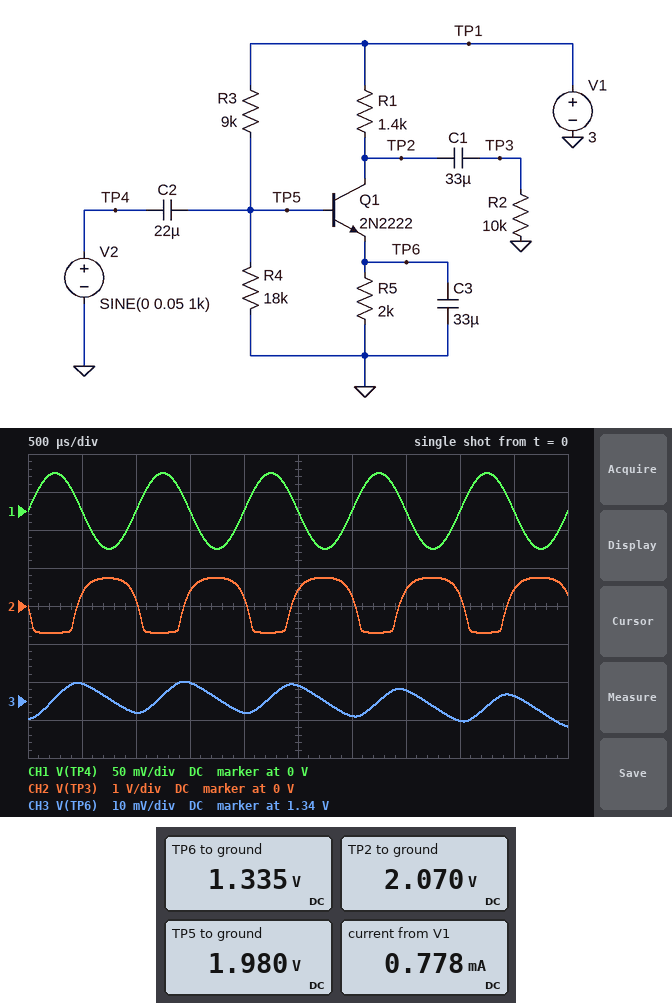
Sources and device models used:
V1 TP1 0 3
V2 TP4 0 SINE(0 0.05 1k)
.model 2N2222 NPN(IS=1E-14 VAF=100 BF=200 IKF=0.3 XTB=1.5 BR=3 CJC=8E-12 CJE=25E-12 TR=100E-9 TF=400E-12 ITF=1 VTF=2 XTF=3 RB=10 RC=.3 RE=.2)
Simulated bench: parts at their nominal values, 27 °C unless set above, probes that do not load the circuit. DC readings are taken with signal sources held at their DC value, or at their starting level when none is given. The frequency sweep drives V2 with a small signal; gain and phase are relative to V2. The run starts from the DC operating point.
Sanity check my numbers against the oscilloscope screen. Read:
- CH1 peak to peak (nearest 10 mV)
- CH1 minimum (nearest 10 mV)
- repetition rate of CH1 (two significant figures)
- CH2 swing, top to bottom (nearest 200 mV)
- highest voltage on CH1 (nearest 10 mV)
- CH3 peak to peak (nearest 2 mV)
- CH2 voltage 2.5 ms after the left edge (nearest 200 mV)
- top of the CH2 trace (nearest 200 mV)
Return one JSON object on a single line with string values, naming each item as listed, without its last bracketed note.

{"CH1 peak to peak": "100 mV", "CH1 minimum": "-50 mV", "repetition rate of CH1": "1.0 kHz", "CH2 swing, top to bottom": "1.4 V", "highest voltage on CH1": "50 mV", "CH3 peak to peak": "12 mV", "CH2 voltage 2.5 ms after the left edge": "400 mV", "top of the CH2 trace": "800 mV"}
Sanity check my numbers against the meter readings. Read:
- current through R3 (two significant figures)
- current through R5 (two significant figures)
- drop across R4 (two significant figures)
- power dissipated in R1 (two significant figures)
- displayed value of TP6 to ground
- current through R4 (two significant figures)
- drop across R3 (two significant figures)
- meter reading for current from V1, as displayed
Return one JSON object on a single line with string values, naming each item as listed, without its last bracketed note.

{"current through R3": "110 µA", "current through R5": "670 µA", "drop across R4": "2.0 V", "power dissipated in R1": "620 µW", "displayed value of TP6 to ground": "1.335 V", "current through R4": "110 µA", "drop across R3": "1.0 V", "meter reading for current from V1, as displayed": "0.778 mA"}
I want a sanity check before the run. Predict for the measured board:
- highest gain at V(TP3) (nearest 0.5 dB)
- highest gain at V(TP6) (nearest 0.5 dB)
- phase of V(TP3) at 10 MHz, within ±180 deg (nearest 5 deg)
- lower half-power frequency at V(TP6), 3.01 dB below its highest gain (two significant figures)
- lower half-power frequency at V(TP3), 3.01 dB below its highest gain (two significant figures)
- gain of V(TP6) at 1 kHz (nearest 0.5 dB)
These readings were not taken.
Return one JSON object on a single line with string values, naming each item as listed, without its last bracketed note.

{"highest gain at V(TP3)": "30.0 dB", "highest gain at V(TP6)": "-0.5 dB", "phase of V(TP3) at 10 MHz, within ±180 deg": "140 deg", "lower half-power frequency at V(TP6), 3.01 dB below its highest gain": "1.2 Hz", "lower half-power frequency at V(TP3), 3.01 dB below its highest gain": "130 Hz", "gain of V(TP6) at 1 kHz": "-18.5 dB"}
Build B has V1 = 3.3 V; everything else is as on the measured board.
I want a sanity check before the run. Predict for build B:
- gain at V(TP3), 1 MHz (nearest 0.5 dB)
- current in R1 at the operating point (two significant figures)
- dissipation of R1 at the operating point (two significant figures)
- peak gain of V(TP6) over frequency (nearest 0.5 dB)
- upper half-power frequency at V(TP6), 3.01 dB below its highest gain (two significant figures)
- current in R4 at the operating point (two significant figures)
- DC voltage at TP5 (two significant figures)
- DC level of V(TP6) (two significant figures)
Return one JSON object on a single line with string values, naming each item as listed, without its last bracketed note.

{"gain at V(TP3), 1 MHz": "31.0 dB", "current in R1 at the operating point": "760 µA", "dissipation of R1 at the operating point": "810 µW", "peak gain of V(TP6) over frequency": "-0.5 dB", "upper half-power frequency at V(TP6), 3.01 dB below its highest gain": "150 Hz", "current in R4 at the operating point": "120 µA", "DC voltage at TP5": "2.2 V", "DC level of V(TP6)": "1.5 V"}
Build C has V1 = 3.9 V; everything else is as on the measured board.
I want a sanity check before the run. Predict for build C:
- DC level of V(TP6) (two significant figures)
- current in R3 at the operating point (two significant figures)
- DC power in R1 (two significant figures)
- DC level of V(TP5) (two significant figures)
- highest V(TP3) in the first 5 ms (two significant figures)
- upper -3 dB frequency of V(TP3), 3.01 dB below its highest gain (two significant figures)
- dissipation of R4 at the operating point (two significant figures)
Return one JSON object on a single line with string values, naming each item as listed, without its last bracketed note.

{"DC level of V(TP6)": "1.9 V", "current in R3 at the operating point": "150 µA", "DC power in R1": "1.3 mW", "DC level of V(TP5)": "2.6 V", "highest V(TP3) in the first 5 ms": "1.1 V", "upper -3 dB frequency of V(TP3), 3.01 dB below its highest gain": "12 MHz", "dissipation of R4 at the operating point": "370 µW"}
